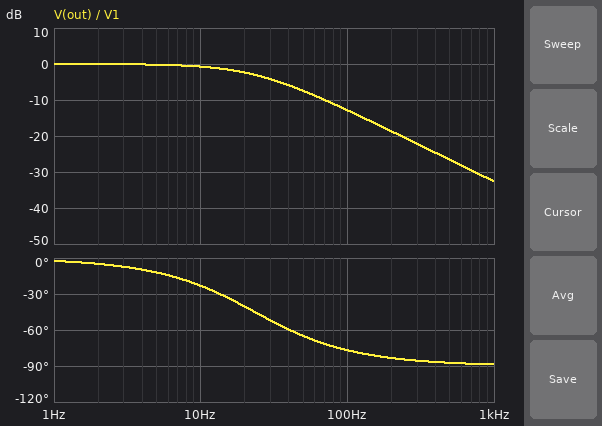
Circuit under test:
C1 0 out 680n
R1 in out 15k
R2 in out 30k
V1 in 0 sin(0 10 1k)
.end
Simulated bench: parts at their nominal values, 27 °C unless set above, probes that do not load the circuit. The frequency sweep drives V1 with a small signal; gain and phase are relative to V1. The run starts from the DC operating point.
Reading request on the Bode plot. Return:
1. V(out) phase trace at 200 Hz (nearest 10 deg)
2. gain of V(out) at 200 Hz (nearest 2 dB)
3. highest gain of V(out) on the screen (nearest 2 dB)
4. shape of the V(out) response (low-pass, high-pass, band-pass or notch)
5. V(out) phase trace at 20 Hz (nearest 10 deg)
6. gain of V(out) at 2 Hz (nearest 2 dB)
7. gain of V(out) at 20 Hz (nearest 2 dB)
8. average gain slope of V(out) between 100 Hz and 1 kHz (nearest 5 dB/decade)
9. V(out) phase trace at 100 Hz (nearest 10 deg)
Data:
-80 deg
-18 dB
0 dB
low-pass
-40 deg
0 dB
-2 dB
-20 dB/decade
-80 deg
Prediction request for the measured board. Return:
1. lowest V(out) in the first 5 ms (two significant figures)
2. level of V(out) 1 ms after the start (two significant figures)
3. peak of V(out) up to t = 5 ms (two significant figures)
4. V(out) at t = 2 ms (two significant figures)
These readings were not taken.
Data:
-120 mV
-32 mV
450 mV
-60 mV
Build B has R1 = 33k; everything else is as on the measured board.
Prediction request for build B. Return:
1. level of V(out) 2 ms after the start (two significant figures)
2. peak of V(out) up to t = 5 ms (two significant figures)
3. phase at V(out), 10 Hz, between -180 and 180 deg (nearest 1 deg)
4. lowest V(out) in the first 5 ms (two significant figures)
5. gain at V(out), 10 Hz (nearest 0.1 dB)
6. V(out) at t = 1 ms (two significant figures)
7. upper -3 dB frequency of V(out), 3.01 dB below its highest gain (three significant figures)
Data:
-25 mV
290 mV
-34 deg
-56 mV
-1.6 dB
-13 mV
14.9 Hz
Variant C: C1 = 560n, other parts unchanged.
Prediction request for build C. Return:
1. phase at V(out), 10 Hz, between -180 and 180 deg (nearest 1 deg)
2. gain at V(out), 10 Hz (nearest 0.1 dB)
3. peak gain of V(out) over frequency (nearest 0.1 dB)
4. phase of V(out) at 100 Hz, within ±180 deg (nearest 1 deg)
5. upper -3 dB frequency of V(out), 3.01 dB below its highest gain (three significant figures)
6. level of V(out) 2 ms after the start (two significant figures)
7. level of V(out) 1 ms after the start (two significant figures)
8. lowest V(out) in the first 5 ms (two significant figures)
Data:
-19 deg
-0.5 dB
0 dB
-74 deg
28.4 Hz
-85 mV
-46 mV
-170 mV
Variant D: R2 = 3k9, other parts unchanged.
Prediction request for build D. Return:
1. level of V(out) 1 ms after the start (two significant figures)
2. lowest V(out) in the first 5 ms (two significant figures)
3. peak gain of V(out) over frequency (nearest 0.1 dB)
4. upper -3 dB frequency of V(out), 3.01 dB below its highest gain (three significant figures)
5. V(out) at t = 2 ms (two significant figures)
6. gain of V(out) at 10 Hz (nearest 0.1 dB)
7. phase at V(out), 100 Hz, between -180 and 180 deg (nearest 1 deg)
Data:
-280 mV
-680 mV
0 dB
75.6 Hz
-460 mV
-0.1 dB
-53 deg
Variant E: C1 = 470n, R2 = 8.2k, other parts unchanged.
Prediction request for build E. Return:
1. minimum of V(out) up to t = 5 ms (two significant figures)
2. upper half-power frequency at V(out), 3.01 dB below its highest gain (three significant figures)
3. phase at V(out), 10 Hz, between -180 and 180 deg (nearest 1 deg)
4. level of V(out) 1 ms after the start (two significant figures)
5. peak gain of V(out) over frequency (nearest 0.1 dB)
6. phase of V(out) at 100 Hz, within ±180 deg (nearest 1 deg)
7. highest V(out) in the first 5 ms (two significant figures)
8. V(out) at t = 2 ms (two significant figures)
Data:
-550 mV
63.9 Hz
-9 deg
-210 mV
0 dB
-57 deg
1.2 V
-350 mV
